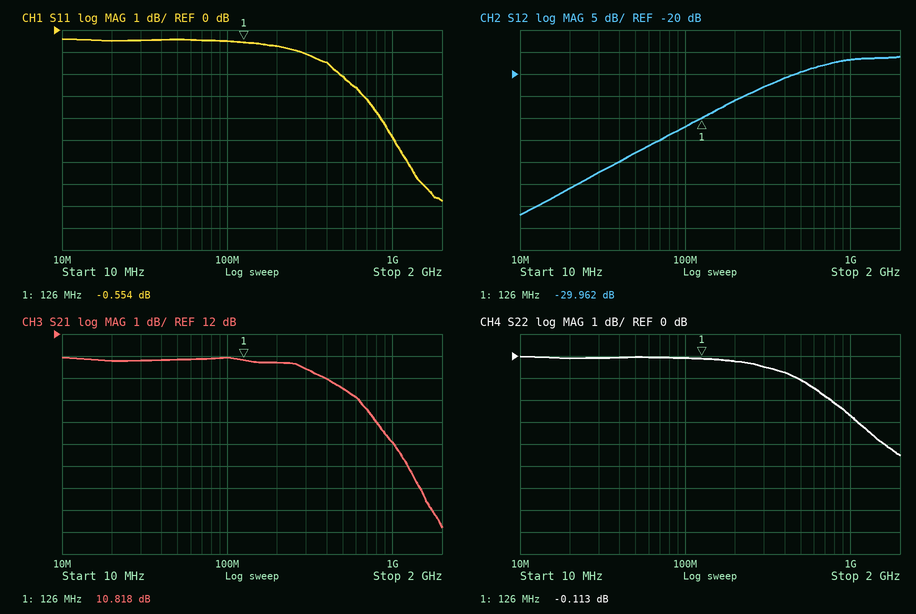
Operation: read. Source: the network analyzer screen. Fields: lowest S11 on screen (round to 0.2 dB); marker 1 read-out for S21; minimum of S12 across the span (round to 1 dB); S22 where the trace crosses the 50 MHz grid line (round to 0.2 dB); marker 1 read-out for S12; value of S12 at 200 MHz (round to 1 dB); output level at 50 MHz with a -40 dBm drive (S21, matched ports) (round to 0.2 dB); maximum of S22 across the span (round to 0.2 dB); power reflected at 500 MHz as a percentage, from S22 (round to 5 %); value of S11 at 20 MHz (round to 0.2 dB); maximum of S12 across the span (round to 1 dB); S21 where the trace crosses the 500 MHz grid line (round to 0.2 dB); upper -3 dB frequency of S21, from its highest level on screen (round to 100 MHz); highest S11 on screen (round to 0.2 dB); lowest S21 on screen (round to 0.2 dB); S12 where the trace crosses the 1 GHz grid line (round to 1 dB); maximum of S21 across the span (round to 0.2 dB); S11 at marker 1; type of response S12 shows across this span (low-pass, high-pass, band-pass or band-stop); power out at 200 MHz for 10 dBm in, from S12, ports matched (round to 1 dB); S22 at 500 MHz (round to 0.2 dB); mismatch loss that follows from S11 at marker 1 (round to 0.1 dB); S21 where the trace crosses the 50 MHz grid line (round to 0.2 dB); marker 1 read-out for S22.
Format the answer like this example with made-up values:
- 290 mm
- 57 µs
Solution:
- -7.8 dB
- 10.818 dB
- -52 dB
- 0.0 dB
- -29.962 dB
- -26 dB
- -29.2 dBm
- 0.0 dB
- 80 %
- -0.4 dB
- -16 dB
- 9.6 dB
- 800 MHz
- -0.4 dB
- 3.2 dB
- -17 dB
- 11.0 dB
- -0.554 dB
- high-pass
- -16 dBm
- -1.0 dB
- 9.2 dB
- 10.8 dB
- -0.113 dB
